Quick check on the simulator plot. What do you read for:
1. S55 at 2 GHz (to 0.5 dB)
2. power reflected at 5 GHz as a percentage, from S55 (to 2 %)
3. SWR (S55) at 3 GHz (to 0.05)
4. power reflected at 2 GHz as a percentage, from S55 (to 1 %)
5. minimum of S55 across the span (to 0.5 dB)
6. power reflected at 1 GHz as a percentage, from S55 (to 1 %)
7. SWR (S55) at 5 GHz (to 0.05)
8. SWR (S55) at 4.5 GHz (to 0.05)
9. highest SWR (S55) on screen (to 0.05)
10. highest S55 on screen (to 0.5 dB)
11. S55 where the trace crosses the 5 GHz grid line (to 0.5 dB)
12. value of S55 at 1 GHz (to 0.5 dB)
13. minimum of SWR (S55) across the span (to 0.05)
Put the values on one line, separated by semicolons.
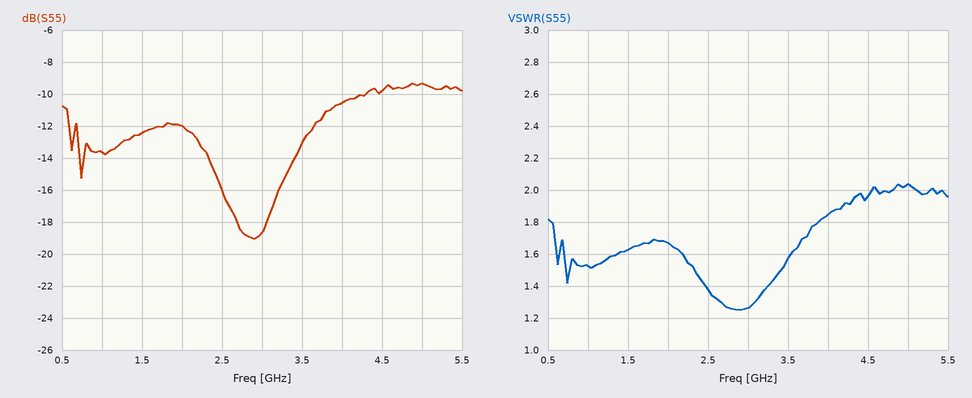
-12.0 dB; 12 %; 1.25; 6 %; -19.0 dB; 4 %; 2.05; 1.95; 2.05; -9.5 dB; -9.5 dB; -13.5 dB; 1.25
